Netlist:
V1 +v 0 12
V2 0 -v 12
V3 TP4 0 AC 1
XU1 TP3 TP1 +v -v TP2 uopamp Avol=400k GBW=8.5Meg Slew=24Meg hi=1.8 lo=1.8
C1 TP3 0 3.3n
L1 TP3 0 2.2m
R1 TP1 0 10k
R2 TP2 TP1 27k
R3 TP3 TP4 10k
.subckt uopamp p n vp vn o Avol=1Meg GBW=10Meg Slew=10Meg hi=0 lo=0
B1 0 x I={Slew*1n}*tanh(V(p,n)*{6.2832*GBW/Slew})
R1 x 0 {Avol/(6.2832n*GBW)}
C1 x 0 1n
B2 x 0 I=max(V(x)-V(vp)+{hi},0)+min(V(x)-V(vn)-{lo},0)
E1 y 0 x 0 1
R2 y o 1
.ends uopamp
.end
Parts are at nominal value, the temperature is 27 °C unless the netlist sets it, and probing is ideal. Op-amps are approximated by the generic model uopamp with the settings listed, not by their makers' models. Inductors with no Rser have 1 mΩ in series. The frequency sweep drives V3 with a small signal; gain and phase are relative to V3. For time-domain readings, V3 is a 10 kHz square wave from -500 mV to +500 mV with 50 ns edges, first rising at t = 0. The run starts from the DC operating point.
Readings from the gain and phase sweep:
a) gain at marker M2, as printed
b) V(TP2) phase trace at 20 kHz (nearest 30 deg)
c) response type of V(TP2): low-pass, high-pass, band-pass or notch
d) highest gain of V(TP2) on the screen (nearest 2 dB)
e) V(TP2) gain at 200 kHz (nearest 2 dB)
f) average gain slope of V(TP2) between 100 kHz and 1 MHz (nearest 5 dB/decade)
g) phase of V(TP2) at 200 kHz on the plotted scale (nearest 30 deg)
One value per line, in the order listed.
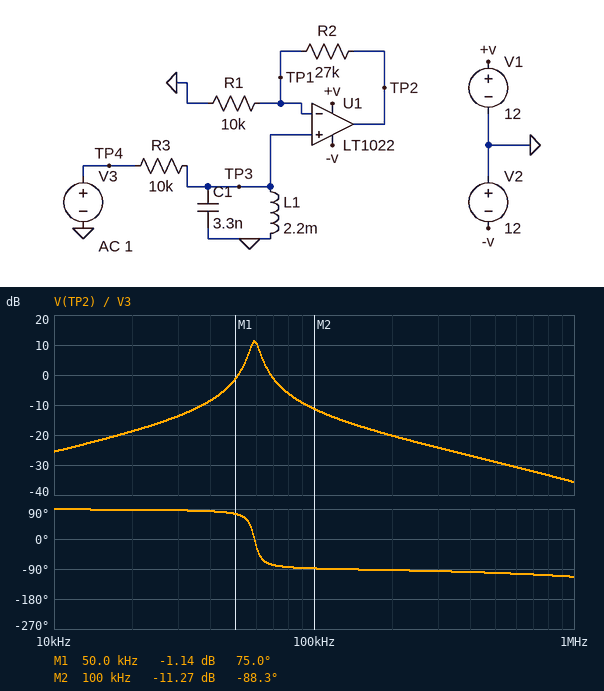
-11.27 dB
90 deg
band-pass
12 dB
-20 dB
-25 dB/decade
-90 deg
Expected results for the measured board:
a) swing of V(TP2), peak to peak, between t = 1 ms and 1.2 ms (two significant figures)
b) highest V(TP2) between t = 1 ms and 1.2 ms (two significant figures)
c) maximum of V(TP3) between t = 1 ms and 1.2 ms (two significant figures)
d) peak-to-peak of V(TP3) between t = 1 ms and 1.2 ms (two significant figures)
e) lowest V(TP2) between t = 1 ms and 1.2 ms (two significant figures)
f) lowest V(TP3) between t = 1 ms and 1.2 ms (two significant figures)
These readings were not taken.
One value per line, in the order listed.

390 mV
200 mV
53 mV
110 mV
-200 mV
-53 mV
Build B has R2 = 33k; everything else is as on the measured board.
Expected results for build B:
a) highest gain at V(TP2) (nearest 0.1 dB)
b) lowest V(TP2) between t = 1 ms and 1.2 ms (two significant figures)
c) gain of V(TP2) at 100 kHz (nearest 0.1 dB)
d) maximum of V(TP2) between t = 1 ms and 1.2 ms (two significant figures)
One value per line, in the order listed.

12.7 dB
-230 mV
-10.0 dB
230 mV
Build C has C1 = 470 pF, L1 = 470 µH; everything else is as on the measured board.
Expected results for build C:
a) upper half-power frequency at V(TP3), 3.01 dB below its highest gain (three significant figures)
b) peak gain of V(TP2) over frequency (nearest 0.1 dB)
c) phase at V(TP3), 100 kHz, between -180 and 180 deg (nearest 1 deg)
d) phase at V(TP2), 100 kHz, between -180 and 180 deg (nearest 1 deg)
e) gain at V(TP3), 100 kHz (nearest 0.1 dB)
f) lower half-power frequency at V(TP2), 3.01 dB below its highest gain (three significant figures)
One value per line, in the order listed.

356 kHz
11.3 dB
88 deg
86 deg
-29.8 dB
322 kHz
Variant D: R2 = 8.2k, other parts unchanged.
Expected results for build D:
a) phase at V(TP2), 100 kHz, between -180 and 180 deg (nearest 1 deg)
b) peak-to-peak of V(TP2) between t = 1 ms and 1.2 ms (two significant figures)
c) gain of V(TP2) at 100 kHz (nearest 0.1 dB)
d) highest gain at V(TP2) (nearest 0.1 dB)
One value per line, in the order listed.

-87 deg
190 mV
-17.4 dB
5.2 dB
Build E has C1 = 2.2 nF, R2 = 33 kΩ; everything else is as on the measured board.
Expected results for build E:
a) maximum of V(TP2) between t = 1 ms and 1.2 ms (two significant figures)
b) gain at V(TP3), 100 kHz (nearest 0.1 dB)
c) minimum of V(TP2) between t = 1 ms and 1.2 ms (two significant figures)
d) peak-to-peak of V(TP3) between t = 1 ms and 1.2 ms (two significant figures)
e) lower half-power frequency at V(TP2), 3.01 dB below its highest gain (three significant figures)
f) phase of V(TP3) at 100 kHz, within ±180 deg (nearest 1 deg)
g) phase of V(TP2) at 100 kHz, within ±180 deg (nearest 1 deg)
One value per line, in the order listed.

520 mV
-16.5 dB
-520 mV
240 mV
68.8 kHz
-81 deg
-84 deg
